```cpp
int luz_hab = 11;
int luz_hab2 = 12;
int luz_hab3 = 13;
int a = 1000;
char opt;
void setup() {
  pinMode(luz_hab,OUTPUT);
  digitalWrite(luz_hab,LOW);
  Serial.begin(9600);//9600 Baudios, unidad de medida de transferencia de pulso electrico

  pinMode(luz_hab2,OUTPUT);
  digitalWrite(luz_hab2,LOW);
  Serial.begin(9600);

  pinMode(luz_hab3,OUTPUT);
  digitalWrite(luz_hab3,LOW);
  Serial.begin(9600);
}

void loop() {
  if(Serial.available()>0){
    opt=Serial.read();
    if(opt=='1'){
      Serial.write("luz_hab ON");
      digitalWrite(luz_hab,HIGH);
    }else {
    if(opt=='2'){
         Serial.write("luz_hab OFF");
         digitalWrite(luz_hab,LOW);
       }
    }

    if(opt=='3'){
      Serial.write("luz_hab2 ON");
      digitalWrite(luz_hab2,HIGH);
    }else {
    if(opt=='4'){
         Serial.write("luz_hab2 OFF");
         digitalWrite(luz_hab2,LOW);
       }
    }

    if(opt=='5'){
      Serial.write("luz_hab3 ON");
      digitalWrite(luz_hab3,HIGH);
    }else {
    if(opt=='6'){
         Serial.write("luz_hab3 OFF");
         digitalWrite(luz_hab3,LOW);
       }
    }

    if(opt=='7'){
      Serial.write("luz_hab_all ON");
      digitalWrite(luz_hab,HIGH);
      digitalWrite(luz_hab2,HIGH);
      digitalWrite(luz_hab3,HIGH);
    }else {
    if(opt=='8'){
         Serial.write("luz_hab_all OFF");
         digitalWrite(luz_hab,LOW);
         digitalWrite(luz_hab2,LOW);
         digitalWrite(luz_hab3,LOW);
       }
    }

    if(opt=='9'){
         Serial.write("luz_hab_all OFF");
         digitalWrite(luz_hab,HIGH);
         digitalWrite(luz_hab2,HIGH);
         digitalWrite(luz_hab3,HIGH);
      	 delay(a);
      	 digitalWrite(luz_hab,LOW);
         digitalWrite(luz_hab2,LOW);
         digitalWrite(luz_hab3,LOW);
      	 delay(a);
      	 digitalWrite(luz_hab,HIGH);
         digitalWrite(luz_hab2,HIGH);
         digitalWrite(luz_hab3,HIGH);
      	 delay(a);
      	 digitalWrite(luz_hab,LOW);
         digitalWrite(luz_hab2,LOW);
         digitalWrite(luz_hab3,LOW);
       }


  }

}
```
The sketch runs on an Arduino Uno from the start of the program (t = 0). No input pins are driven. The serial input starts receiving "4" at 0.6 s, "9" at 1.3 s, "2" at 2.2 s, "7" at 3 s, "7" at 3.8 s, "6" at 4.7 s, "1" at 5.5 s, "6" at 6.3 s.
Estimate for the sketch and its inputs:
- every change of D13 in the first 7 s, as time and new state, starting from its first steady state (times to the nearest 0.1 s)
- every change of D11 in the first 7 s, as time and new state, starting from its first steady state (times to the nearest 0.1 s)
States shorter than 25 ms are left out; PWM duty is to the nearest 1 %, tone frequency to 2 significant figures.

0 s low; 1.3 s high; 2.3 s low; 3.3 s high; 4.7 s low
0 s low; 1.3 s high; 2.3 s low; 3.3 s high
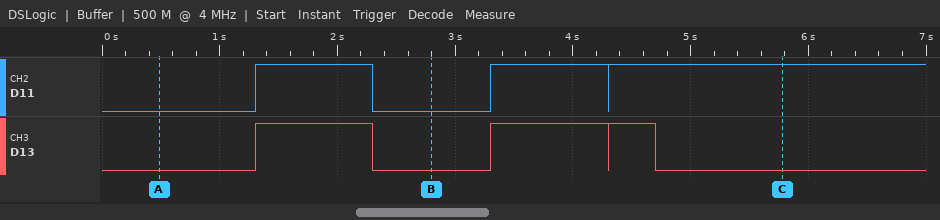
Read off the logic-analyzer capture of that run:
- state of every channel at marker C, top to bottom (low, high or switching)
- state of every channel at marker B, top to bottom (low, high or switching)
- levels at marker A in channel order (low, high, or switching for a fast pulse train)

D11 high, D13 low
D11 low, D13 low
D11 low, D13 low
